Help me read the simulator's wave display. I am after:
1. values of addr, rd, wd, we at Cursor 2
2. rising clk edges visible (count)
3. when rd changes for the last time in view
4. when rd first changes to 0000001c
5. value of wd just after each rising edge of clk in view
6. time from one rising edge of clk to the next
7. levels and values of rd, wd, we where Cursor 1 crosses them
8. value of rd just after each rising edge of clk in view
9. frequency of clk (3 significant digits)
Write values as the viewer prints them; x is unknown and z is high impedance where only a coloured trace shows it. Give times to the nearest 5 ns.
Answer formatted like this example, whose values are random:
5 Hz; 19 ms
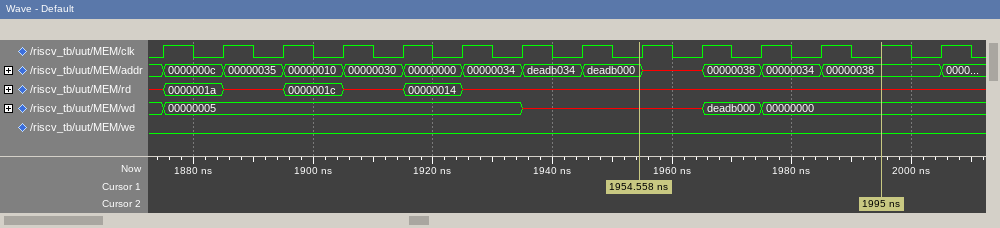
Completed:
addr=00000038, rd=x, wd=00000000, we=0; 14; 1925 ns; 1895 ns; 00000005, 00000005, 00000005, 00000005, 00000005, 00000005, x, x, x, deadb000, 00000000, 00000000, 00000000, 00000000; 10 ns; rd=x, wd=x, we=0; 0000001a, x, 0000001c, x, 00000014, x, x, x, x, x, x, x, x, x; 100 MHz
